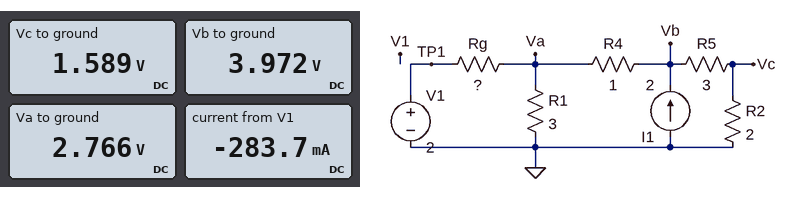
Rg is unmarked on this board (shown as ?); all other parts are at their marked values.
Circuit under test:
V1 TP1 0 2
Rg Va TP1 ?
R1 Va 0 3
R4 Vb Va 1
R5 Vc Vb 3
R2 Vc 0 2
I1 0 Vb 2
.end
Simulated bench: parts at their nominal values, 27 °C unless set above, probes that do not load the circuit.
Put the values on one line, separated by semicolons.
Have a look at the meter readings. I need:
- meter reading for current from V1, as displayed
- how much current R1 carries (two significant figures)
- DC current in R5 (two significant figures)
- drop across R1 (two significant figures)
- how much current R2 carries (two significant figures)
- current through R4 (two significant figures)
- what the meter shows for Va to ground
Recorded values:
-283.7 mA; 920 mA; 790 mA; 2.8 V; 790 mA; 1.2 A; 2.766 V
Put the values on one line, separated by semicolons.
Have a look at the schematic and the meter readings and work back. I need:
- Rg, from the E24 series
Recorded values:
2.7 Ω
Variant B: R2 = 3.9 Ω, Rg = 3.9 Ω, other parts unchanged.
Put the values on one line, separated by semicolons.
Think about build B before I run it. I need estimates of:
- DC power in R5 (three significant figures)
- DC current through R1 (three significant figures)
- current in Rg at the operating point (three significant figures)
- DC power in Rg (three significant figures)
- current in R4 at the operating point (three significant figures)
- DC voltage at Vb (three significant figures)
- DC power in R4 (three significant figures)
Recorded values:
1.28 W; 1.05 A; 296 mA; 342 mW; 1.35 A; 4.50 V; 1.82 W
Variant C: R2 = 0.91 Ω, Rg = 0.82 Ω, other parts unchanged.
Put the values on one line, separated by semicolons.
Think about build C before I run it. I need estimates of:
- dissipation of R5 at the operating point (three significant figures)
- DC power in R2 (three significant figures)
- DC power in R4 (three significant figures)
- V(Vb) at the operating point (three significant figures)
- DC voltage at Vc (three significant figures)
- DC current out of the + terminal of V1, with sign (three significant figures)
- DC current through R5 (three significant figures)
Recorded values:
2.30 W; 696 mW; 1.27 W; 3.42 V; 796 mV; -360 mA; 875 mA
